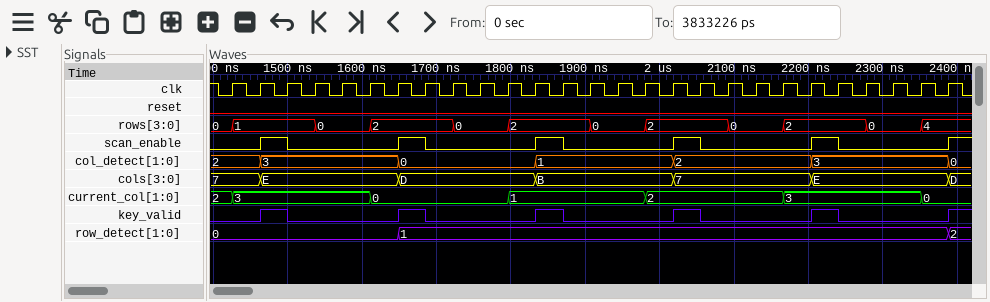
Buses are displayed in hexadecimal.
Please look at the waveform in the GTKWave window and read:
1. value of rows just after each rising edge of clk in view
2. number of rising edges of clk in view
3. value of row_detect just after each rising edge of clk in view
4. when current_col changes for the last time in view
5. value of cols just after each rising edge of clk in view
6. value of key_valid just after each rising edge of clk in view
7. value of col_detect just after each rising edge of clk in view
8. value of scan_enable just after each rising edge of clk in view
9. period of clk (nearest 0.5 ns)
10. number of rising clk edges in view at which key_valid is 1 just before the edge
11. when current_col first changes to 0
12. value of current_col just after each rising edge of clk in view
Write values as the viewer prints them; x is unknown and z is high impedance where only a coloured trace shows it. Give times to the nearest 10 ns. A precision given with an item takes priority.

1, 1, 1, 0, 0, 2, 2, 2, 0, 0, 2, 2, 2, 0, 0, 2, 2, 2, 0, 0, 2, 2, 2, 0, 0, 4, 4
27
0, 0, 0, 0, 0, 0, 1, 1, 1, 1, 1, 1, 1, 1, 1, 1, 1, 1, 1, 1, 1, 1, 1, 1, 1, 1, 2
2350 ns
7, E, E, E, E, E, D, D, D, D, D, B, B, B, B, B, 7, 7, 7, 7, 7, E, E, E, E, E, D
0 1 0 0 0 0 1 0 0 0 0 1 0 0 0 0 1 0 0 0 0 1 0 0 0 0 1
2, 3, 3, 3, 3, 3, 0, 0, 0, 0, 0, 1, 1, 1, 1, 1, 2, 2, 2, 2, 2, 3, 3, 3, 3, 3, 0
0 1 0 0 0 0 1 0 0 0 0 1 0 0 0 0 1 0 0 0 0 1 0 0 0 0 1
37 ns
5
1610 ns
3, 3, 3, 3, 3, 0, 0, 0, 0, 0, 1, 1, 1, 1, 1, 2, 2, 2, 2, 2, 3, 3, 3, 3, 3, 0, 0
